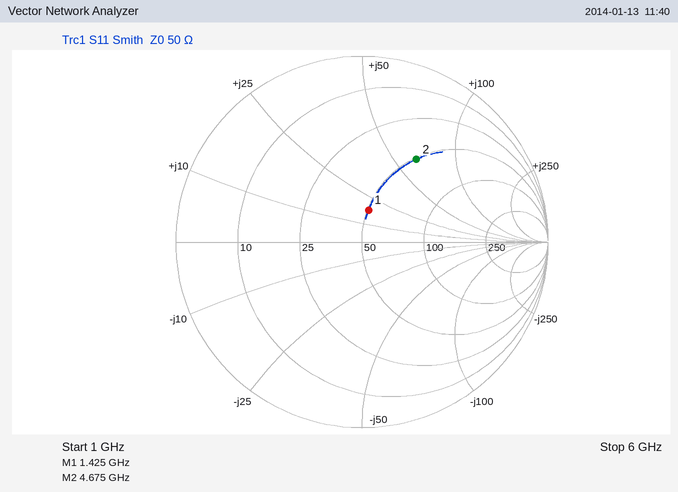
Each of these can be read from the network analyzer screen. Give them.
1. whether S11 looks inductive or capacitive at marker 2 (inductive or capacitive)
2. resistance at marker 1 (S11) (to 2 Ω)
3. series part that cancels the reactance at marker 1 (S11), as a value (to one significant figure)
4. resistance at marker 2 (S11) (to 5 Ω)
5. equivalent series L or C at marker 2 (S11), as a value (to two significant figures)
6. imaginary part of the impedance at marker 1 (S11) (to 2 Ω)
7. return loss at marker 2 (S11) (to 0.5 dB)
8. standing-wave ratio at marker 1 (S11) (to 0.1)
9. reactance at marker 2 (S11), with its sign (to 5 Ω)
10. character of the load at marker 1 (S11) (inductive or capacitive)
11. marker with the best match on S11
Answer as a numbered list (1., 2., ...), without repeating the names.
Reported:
1. inductive
2. 50 Ω
3. 6 pF
4. 50 Ω
5. 2.2 nH
6. +18 Ω
7. 5.5 dB
8. 1.4
9. +65 Ω
10. inductive
11. marker 1
